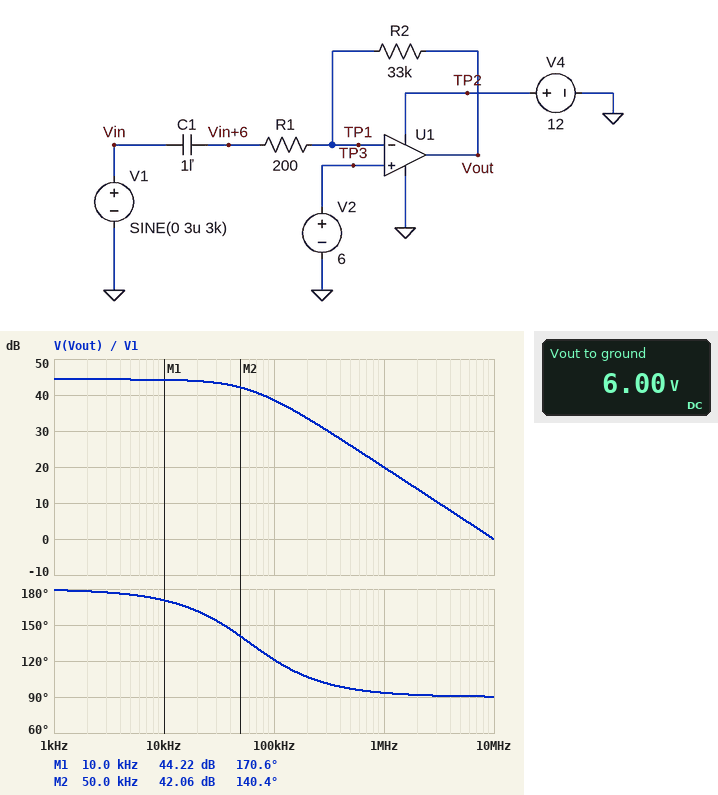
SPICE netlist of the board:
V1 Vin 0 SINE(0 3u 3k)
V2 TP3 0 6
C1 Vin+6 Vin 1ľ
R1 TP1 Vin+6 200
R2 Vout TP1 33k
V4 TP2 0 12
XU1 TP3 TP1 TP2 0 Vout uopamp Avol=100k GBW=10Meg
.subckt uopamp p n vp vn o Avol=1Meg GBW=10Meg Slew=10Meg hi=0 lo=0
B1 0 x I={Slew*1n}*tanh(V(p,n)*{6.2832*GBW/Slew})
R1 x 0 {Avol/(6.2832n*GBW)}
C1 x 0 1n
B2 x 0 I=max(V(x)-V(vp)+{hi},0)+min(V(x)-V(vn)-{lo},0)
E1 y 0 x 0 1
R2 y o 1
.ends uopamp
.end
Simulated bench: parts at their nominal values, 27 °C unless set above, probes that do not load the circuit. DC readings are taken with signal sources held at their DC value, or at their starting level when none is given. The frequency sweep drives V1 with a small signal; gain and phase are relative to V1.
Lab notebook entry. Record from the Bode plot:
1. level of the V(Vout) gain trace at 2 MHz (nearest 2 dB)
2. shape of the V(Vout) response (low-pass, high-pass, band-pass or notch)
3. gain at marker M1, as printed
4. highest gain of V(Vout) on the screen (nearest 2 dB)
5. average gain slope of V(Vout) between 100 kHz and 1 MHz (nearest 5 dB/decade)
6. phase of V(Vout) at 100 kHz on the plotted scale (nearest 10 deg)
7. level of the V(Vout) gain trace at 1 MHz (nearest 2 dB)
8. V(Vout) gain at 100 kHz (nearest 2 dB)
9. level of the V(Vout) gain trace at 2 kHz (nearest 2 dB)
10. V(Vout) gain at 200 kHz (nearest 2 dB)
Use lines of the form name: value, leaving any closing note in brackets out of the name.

level of the V(Vout) gain trace at 2 MHz: 14 dB
shape of the V(Vout) response: low-pass
gain at marker M1, as printed: 44.22 dB
highest gain of V(Vout) on the screen: 44 dB
average gain slope of V(Vout) between 100 kHz and 1 MHz: -20 dB/decade
phase of V(Vout) at 100 kHz on the plotted scale: 120 deg
level of the V(Vout) gain trace at 1 MHz: 20 dB
V(Vout) gain at 100 kHz: 38 dB
level of the V(Vout) gain trace at 2 kHz: 44 dB
V(Vout) gain at 200 kHz: 34 dB
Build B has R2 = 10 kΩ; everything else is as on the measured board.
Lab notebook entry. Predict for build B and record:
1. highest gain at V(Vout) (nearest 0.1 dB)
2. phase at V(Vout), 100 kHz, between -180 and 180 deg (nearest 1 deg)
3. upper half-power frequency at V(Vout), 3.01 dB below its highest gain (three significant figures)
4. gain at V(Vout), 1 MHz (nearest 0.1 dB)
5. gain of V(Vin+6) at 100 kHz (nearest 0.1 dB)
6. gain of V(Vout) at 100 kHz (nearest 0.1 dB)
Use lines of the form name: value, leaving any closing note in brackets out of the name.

highest gain at V(Vout): 34.0 dB
phase at V(Vout), 100 kHz, between -180 and 180 deg: 153 deg
upper half-power frequency at V(Vout), 3.01 dB below its highest gain: 196 kHz
gain at V(Vout), 1 MHz: 19.7 dB
gain of V(Vin+6) at 100 kHz: 0 dB
gain of V(Vout) at 100 kHz: 33.0 dB
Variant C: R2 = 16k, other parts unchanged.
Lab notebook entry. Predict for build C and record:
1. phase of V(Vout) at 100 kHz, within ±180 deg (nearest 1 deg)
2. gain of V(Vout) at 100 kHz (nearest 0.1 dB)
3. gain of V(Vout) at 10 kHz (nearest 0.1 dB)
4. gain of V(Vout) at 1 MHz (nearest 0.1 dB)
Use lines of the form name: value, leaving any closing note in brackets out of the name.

phase of V(Vout) at 100 kHz, within ±180 deg: 141 deg
gain of V(Vout) at 100 kHz: 35.9 dB
gain of V(Vout) at 10 kHz: 38.0 dB
gain of V(Vout) at 1 MHz: 19.8 dB
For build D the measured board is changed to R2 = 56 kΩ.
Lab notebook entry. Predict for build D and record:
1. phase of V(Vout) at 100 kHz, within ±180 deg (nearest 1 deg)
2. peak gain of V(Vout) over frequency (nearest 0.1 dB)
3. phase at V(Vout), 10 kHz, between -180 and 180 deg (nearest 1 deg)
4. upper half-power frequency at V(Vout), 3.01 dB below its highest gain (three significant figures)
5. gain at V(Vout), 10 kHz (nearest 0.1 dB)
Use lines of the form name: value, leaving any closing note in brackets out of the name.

phase of V(Vout) at 100 kHz, within ±180 deg: 110 deg
peak gain of V(Vout) over frequency: 48.9 dB
phase at V(Vout), 10 kHz, between -180 and 180 deg: 164 deg
upper half-power frequency at V(Vout), 3.01 dB below its highest gain: 35.7 kHz
gain at V(Vout), 10 kHz: 48.6 dB
